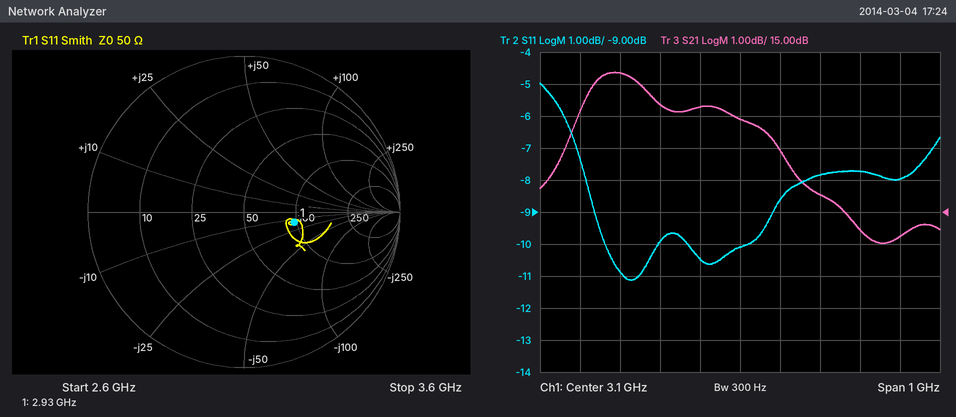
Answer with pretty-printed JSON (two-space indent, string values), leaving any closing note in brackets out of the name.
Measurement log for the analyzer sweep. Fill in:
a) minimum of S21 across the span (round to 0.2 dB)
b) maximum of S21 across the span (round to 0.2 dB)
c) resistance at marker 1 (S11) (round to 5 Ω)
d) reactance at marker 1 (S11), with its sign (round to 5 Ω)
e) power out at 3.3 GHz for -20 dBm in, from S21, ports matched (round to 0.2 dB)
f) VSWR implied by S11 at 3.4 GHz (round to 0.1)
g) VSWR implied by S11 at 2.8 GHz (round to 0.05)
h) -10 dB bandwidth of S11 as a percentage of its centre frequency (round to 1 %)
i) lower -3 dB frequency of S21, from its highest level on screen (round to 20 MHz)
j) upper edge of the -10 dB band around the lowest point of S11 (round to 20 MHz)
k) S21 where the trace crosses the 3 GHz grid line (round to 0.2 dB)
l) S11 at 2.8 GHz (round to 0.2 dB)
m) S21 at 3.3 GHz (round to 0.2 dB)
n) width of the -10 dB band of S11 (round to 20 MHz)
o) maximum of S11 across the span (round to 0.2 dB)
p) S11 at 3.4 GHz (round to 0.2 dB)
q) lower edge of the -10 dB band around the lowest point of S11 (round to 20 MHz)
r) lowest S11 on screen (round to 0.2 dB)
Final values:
{
  "minimum of S21 across the span": "14.0 dB",
  "maximum of S21 across the span": "19.4 dB",
  "resistance at marker 1 (S11)": "95 Ω",
  "reactance at marker 1 (S11), with its sign": "-15 Ω",
  "power out at 3.3 GHz for -20 dBm in, from S21, ports matched": "-4.4 dBm",
  "VSWR implied by S11 at 3.4 GHz": "2.4",
  "VSWR implied by S11 at 2.8 GHz": "1.80",
  "-10 dB bandwidth of S11 as a percentage of its centre frequency": "5 %",
  "lower -3 dB frequency of S21, from its highest level on screen": "2.64 GHz",
  "upper edge of the -10 dB band around the lowest point of S11": "2.90 GHz",
  "S21 where the trace crosses the 3 GHz grid line": "18.2 dB",
  "S11 at 2.8 GHz": "-10.8 dB",
  "S21 at 3.3 GHz": "15.6 dB",
  "width of the -10 dB band of S11": "140 MHz",
  "maximum of S11 across the span": "-5.0 dB",
  "S11 at 3.4 GHz": "-7.8 dB",
  "lower edge of the -10 dB band around the lowest point of S11": "2.76 GHz",
  "lowest S11 on screen": "-11.2 dB"
}
